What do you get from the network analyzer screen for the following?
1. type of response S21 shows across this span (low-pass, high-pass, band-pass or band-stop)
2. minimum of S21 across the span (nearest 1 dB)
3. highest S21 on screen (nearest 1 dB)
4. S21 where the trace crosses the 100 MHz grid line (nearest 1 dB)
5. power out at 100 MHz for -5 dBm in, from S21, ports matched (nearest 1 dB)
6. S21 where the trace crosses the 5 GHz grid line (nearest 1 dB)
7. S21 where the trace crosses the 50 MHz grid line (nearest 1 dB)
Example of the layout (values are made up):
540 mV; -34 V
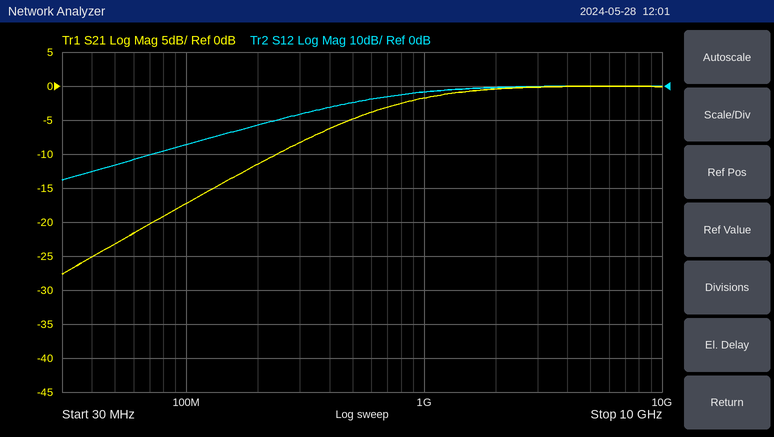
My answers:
high-pass; -28 dB; 0 dB; -17 dB; -22 dBm; 0 dB; -23 dB
